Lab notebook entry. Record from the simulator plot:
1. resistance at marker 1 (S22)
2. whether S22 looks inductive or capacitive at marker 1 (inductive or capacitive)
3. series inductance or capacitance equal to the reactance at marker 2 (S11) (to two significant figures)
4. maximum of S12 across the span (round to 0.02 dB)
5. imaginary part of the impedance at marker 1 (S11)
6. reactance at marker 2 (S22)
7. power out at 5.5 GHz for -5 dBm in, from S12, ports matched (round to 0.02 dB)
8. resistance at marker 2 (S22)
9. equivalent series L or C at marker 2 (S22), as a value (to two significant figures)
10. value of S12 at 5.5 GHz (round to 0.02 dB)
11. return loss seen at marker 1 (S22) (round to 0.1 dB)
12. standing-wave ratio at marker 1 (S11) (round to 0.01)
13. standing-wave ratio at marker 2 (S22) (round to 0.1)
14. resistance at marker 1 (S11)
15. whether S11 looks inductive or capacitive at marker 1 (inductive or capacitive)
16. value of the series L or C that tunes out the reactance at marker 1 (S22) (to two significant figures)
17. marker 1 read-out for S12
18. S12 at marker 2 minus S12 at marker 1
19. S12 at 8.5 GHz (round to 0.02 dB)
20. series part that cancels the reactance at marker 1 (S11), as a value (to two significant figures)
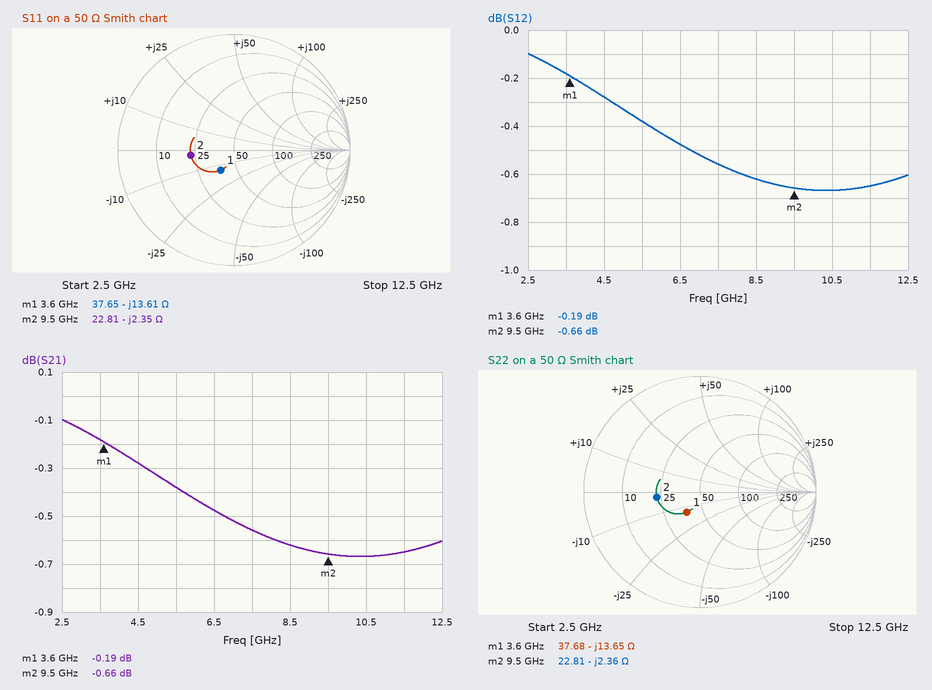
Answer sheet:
37.68 Ω
capacitive
7.1 pF
-0.10 dB
-13.61 Ω
-2.36 Ω
-5.38 dBm
22.81 Ω
7.1 pF
-0.38 dB
13.7 dB
1.52
2.2
37.65 Ω
capacitive
600 pH
-0.19 dB
-0.47 dB
-0.62 dB
600 pH
